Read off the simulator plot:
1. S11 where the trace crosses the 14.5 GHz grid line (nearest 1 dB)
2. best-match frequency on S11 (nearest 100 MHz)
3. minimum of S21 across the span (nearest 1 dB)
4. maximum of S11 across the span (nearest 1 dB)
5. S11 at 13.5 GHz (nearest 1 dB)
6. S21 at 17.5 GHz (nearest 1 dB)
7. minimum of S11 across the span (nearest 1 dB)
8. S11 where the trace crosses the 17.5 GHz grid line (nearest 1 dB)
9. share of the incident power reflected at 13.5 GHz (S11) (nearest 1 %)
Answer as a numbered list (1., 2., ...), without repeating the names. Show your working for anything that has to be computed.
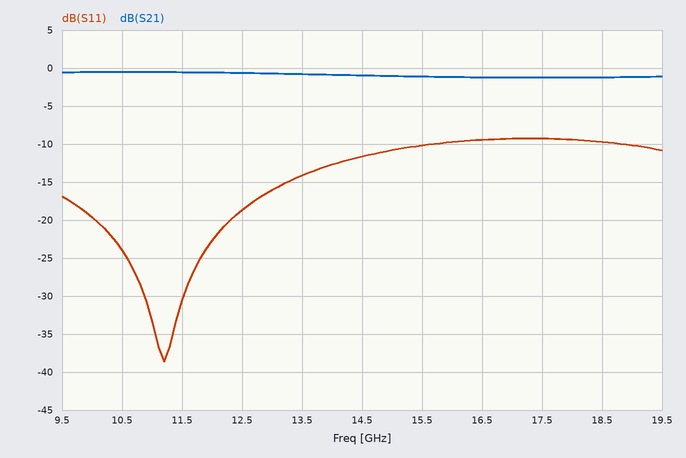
1. -12 dB
2. 11.2 GHz
3. -1 dB
4. -9 dB
5. -14 dB
6. -1 dB
7. -39 dB
8. -9 dB
9. 10^(-14/10) ≈ 4 %
